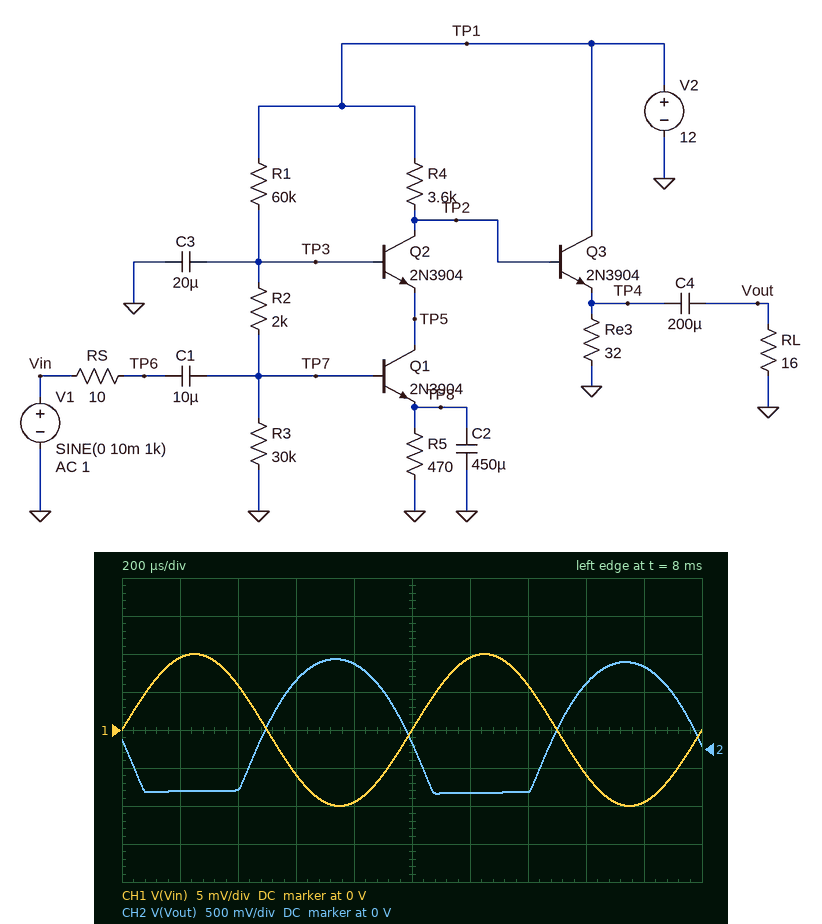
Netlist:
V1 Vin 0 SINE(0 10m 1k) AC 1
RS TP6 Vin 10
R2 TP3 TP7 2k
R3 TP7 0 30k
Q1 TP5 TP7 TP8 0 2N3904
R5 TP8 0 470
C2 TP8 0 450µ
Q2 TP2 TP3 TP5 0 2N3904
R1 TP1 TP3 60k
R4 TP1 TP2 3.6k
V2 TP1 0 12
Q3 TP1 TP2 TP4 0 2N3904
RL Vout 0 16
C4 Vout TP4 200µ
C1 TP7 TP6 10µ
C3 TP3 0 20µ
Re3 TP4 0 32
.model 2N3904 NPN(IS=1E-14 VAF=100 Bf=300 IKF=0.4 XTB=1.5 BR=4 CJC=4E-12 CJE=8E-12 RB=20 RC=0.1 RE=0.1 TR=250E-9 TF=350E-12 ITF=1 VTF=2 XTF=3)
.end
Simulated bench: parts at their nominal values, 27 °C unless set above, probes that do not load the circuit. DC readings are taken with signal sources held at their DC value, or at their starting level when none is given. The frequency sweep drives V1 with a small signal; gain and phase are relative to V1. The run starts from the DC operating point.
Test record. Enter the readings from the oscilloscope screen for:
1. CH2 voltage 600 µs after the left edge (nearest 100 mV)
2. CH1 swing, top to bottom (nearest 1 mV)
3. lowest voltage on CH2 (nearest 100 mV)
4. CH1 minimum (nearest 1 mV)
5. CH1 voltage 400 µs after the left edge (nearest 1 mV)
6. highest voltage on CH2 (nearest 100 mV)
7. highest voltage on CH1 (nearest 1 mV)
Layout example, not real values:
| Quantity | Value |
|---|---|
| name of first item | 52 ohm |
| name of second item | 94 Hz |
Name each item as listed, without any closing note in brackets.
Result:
| Quantity | Value |
|---|---|
| CH2 voltage 600 µs after the left edge | 900 mV |
| CH1 swing, top to bottom | 20 mV |
| lowest voltage on CH2 | -600 mV |
| CH1 minimum | -10 mV |
| CH1 voltage 400 µs after the left edge | 6 mV |
| highest voltage on CH2 | 1.2 V |
| highest voltage on CH1 | 10 mV |
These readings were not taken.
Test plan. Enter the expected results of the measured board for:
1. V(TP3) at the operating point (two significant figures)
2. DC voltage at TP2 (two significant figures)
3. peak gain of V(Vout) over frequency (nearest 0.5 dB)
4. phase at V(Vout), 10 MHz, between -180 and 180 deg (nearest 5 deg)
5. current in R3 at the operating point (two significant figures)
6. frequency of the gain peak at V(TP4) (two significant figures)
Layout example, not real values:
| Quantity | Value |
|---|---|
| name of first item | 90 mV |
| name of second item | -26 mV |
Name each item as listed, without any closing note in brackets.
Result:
| Quantity | Value |
|---|---|
| V(TP3) at the operating point | 2.2 V |
| DC voltage at TP2 | 1.6 V |
| peak gain of V(Vout) over frequency | 31.0 dB |
| phase at V(Vout), 10 MHz, between -180 and 180 deg | 120 deg |
| current in R3 at the operating point | 68 µA |
| frequency of the gain peak at V(TP4) | 100 Hz |
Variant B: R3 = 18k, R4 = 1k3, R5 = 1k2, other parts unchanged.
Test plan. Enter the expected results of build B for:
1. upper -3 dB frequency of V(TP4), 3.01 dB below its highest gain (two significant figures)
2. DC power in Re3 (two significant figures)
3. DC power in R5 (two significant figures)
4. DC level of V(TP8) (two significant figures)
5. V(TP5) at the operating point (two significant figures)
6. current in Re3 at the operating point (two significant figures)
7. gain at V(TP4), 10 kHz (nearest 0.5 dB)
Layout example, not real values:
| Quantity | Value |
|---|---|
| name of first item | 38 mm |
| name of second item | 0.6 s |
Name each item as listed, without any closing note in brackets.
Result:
| Quantity | Value |
|---|---|
| upper -3 dB frequency of V(TP4), 3.01 dB below its highest gain | 4.8 MHz |
| DC power in Re3 | 1.8 W |
| DC power in R5 | 3.0 mW |
| DC level of V(TP8) | 1.9 V |
| V(TP5) at the operating point | 2.2 V |
| current in Re3 at the operating point | 240 mA |
| gain at V(TP4), 10 kHz | 32.0 dB |
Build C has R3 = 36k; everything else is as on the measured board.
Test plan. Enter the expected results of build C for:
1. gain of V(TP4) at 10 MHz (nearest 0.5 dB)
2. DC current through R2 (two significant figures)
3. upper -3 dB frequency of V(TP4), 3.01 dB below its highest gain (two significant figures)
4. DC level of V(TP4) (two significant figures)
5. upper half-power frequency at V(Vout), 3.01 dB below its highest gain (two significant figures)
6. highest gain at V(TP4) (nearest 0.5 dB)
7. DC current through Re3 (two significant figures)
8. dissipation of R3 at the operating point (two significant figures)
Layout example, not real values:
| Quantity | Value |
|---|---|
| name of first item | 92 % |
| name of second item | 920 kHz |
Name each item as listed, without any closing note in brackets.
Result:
| Quantity | Value |
|---|---|
| gain of V(TP4) at 10 MHz | 0.5 dB |
| DC current through R2 | 71 µA |
| upper -3 dB frequency of V(TP4), 3.01 dB below its highest gain | 92 kHz |
| DC level of V(TP4) | 830 mV |
| upper half-power frequency at V(Vout), 3.01 dB below its highest gain | 130 kHz |
| highest gain at V(TP4) | 30.0 dB |
| DC current through Re3 | 26 mA |
| dissipation of R3 at the operating point | 120 µW |
